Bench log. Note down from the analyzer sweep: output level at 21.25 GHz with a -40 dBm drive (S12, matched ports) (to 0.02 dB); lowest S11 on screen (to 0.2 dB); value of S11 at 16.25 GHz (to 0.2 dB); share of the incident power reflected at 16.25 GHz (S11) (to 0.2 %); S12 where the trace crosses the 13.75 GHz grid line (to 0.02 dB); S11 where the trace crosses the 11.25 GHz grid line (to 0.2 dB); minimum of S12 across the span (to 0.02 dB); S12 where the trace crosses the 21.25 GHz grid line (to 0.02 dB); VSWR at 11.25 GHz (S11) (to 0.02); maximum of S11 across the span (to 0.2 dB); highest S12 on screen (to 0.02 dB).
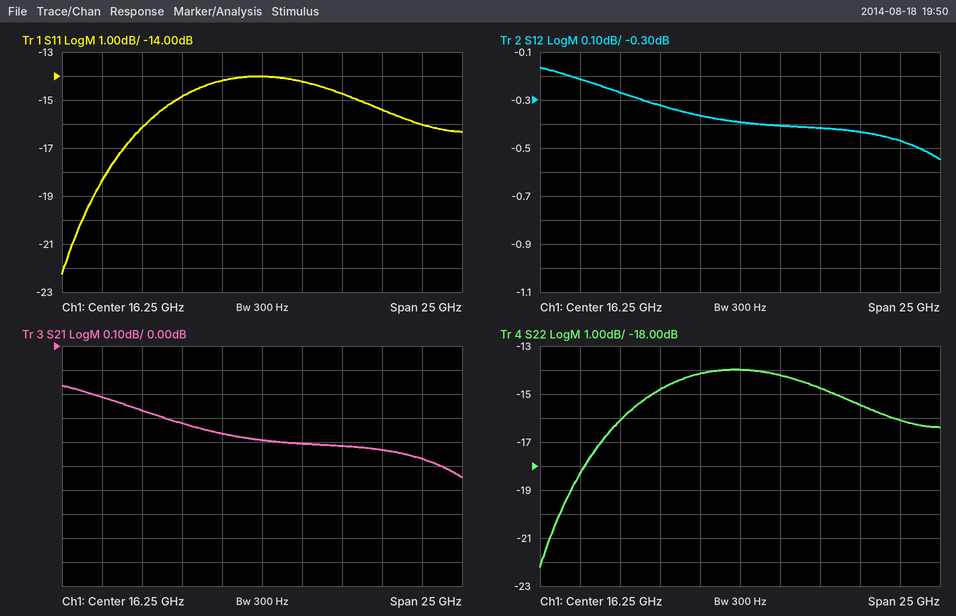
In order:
-40.42 dBm
-22.2 dB
-14.0 dB
4.0 %
-0.36 dB
-14.8 dB
-0.54 dB
-0.42 dB
1.44
-14.0 dB
-0.16 dB
